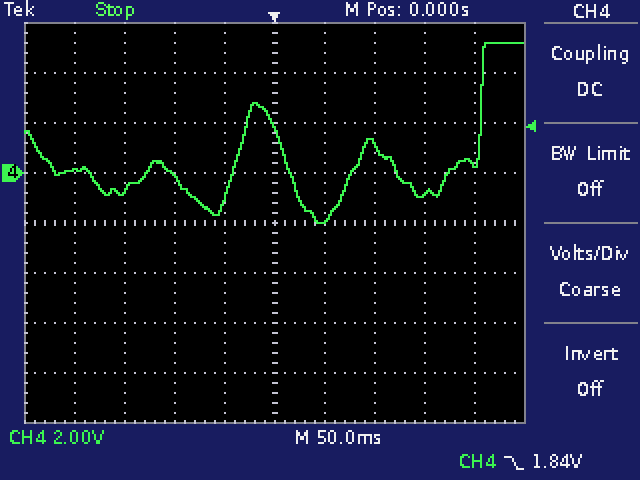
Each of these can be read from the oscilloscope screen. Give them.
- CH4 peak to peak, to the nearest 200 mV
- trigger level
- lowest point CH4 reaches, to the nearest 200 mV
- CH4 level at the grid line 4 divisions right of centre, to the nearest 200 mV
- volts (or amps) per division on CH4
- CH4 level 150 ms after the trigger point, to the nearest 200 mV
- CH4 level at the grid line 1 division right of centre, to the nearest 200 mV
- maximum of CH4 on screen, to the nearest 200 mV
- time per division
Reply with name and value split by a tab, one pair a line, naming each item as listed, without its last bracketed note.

CH4 peak to peak, to the nearest 200 mV	7.2 V
trigger level	1.84 V
lowest point CH4 reaches, to the nearest 200 mV	-2.0 V
CH4 level at the grid line 4 divisions right of centre, to the nearest 200 mV	400 mV
volts (or amps) per division on CH4	2 V
CH4 level 150 ms after the trigger point, to the nearest 200 mV	-800 mV
CH4 level at the grid line 1 division right of centre, to the nearest 200 mV	-2.0 V
maximum of CH4 on screen, to the nearest 200 mV	5.2 V
time per division	50 ms
